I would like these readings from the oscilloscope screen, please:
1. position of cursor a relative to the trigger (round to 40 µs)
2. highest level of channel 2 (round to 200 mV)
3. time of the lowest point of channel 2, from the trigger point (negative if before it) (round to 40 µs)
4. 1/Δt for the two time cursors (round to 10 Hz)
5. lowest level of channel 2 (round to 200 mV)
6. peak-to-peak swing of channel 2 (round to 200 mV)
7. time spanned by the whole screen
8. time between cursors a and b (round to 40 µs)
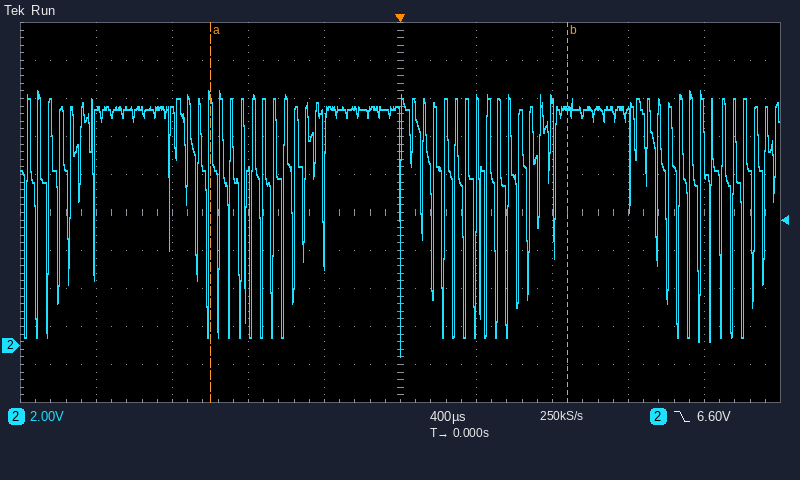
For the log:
-1.00 ms
13.4 V
0 µs
530 Hz
-600 mV
14.0 V
4 ms
1.88 ms
